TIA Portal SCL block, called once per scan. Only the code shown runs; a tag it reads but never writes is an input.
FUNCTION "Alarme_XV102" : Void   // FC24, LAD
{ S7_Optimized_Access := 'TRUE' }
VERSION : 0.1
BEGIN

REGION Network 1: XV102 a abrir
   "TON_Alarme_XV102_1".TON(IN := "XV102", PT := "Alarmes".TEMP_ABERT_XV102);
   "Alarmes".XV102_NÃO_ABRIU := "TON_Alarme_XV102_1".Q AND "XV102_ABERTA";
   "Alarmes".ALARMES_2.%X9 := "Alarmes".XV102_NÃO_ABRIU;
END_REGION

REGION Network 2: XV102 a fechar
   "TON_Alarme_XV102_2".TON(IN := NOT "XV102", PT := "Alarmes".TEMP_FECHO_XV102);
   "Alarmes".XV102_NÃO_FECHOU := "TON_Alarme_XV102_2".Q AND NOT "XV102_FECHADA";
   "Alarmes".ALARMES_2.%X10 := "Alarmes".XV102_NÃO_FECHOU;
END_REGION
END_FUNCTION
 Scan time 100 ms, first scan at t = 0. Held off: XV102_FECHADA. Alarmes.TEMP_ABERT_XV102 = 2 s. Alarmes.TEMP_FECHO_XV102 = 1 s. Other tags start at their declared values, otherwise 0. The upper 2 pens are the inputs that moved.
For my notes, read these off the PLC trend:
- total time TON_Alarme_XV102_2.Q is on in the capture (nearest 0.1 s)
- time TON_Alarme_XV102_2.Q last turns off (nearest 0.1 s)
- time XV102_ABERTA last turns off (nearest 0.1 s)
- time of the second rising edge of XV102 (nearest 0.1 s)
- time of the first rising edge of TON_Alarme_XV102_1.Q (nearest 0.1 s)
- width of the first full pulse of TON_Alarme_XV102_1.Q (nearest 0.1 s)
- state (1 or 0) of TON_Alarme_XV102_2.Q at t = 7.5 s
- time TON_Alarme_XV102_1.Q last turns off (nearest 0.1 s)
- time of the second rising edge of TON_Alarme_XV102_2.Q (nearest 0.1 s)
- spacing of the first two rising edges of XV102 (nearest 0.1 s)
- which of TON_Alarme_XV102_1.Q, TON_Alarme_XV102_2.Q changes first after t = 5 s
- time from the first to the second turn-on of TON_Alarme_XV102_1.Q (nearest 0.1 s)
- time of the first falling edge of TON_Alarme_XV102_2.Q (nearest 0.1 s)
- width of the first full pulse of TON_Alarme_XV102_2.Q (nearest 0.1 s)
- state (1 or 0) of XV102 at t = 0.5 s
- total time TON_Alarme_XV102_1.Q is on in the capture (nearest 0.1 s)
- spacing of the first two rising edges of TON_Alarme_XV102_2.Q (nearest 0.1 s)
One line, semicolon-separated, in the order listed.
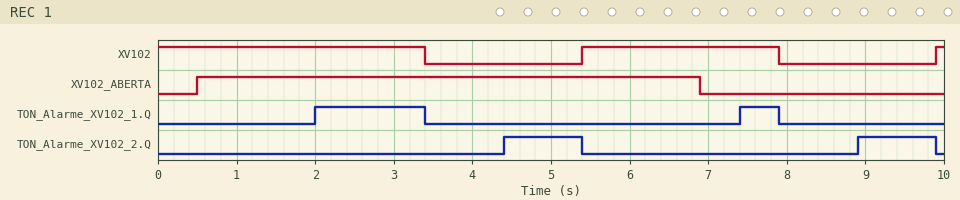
2.0 s; 9.9 s; 6.9 s; 9.9 s; 2.0 s; 1.4 s; 0; 7.9 s; 8.9 s; 4.5 s; TON_Alarme_XV102_2.Q; 5.4 s; 5.4 s; 1.0 s; 1; 1.9 s; 4.5 s
